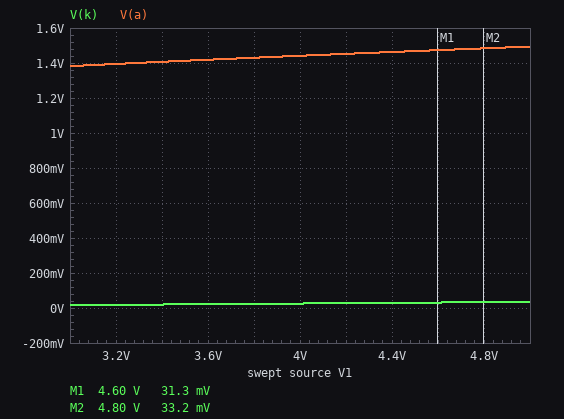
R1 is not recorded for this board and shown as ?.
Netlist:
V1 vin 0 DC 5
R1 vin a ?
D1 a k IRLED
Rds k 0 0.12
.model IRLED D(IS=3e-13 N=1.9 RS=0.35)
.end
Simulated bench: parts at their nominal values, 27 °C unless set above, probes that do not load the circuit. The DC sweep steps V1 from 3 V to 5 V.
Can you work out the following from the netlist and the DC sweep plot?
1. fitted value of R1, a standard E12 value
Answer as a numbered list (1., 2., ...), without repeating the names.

1. 12 Ω
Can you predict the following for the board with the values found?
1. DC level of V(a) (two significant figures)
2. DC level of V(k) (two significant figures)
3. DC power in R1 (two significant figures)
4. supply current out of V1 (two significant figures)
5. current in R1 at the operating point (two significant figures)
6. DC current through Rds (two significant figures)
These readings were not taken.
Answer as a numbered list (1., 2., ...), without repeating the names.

1. 1.5 V
2. 35 mV
3. 1.0 W
4. 290 mA
5. 290 mA
6. 290 mA
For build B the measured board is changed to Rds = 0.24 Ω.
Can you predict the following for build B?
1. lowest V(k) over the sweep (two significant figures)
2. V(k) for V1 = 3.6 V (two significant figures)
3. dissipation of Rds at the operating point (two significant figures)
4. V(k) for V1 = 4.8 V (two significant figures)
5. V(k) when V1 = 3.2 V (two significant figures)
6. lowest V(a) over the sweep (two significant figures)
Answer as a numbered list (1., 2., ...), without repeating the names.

1. 32 mV
2. 43 mV
3. 20 mW
4. 66 mV
5. 36 mV
6. 1.4 V
